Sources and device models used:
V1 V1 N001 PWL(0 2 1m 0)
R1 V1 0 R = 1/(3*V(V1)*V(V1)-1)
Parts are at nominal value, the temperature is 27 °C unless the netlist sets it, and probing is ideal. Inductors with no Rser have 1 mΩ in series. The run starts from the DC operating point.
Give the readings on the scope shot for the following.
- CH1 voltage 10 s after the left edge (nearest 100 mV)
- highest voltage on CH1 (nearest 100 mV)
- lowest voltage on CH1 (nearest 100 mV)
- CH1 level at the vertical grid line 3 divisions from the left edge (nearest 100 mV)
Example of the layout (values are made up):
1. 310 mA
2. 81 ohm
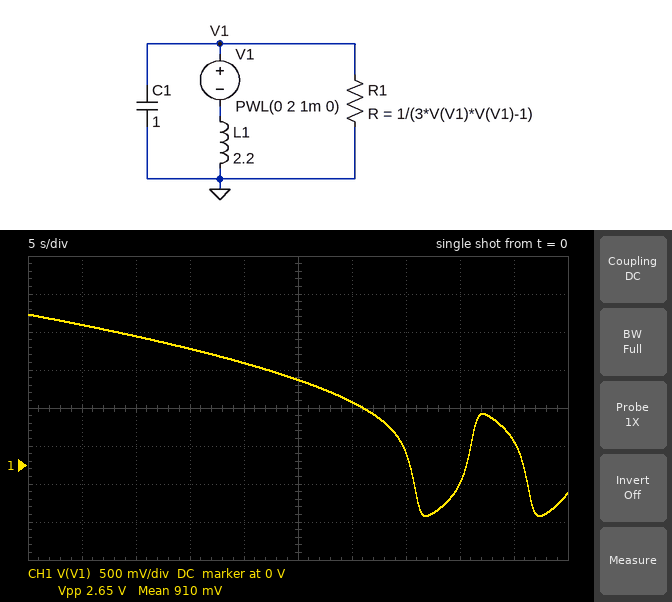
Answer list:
1. 1.7 V
2. 2.0 V
3. -700 mV
4. 1.5 V
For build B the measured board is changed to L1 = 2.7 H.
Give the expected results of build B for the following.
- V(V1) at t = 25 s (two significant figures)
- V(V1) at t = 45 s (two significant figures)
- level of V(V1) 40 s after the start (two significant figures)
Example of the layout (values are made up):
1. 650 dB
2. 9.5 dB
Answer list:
1. 1.3 V
2. -670 mV
3. 600 mV
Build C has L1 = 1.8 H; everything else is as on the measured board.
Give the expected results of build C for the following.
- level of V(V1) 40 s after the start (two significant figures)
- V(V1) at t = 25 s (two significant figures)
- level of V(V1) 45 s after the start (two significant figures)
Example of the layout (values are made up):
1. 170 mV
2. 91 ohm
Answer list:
1. -670 mV
2. 790 mV
3. 640 mV
